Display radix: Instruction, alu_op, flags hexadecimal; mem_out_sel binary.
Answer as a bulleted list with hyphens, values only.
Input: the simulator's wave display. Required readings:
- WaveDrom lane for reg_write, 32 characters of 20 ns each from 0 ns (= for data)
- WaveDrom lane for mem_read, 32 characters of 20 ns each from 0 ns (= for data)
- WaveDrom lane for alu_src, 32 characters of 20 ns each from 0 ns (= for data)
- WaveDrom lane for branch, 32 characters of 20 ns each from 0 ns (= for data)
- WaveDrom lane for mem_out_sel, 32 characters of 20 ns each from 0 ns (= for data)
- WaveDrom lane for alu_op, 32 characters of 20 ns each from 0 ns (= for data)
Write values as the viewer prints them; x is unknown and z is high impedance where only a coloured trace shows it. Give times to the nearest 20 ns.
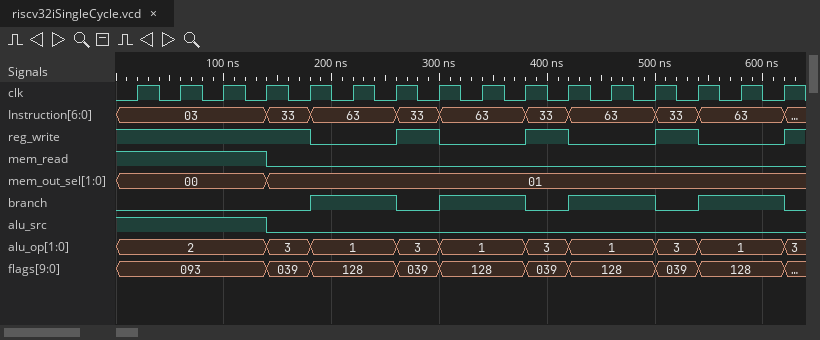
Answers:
- {name: 'reg_write', wave: '1........0...1.0...1.0...1.0...1'}
- {name: 'mem_read', wave: '1......0........................'}
- {name: 'alu_src', wave: '1......0........................'}
- {name: 'branch', wave: '0........1...0.1...0.1...0.1...0'}
- {name: 'mem_out_sel', wave: '=......=........................', data: '00 01'}
- {name: 'alu_op', wave: '=......=.=...=.=...=.=...=.=...=', data: '2 3 1 3 1 3 1 3 1 3'}
